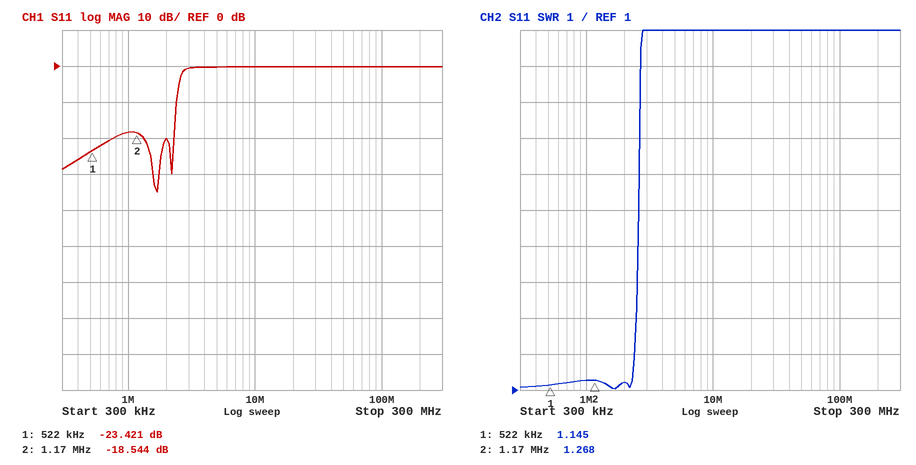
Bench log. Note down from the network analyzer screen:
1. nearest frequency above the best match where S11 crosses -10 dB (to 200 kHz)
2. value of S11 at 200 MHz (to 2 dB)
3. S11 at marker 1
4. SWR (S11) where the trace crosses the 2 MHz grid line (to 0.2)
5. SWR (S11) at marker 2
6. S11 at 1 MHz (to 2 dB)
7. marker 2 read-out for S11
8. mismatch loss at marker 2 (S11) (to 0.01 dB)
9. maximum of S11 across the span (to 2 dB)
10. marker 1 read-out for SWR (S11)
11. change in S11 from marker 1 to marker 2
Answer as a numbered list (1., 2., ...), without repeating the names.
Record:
1. 2.4 MHz
2. 0 dB
3. -23.421 dB
4. 1.2
5. 1.268
6. -18 dB
7. -18.544 dB
8. 0.06 dB
9. 0 dB
10. 1.145
11. 4.877 dB
